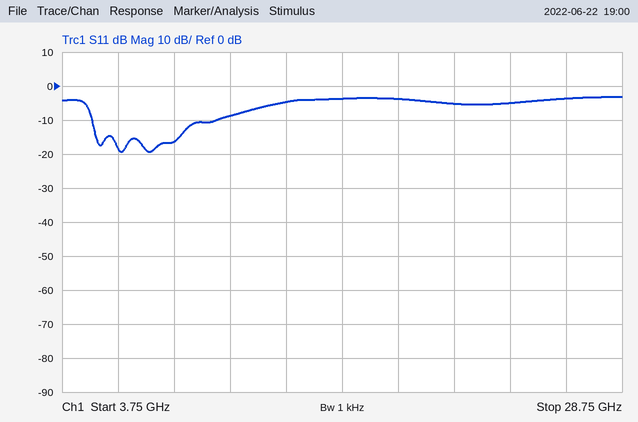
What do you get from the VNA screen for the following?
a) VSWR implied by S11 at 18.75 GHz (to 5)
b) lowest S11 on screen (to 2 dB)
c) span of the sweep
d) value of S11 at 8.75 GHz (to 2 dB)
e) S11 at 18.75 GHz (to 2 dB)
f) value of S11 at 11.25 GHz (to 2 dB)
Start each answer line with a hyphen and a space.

- 5
- -20 dB
- 25 GHz
- -16 dB
- -4 dB
- -8 dB
